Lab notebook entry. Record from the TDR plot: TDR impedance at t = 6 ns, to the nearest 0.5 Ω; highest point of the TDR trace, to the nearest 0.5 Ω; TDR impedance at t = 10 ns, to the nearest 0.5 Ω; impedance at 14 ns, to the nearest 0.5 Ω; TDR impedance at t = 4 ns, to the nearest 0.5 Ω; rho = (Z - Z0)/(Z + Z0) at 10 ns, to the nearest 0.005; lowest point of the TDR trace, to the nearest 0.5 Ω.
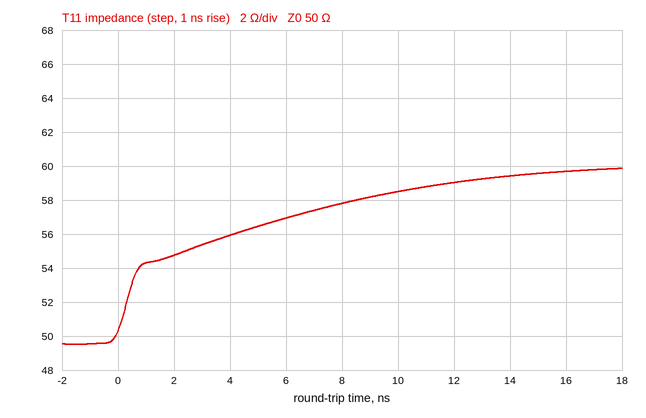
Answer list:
57.0 Ω
60.0 Ω
58.5 Ω
59.5 Ω
56.0 Ω
+0.080
49.5 Ω
